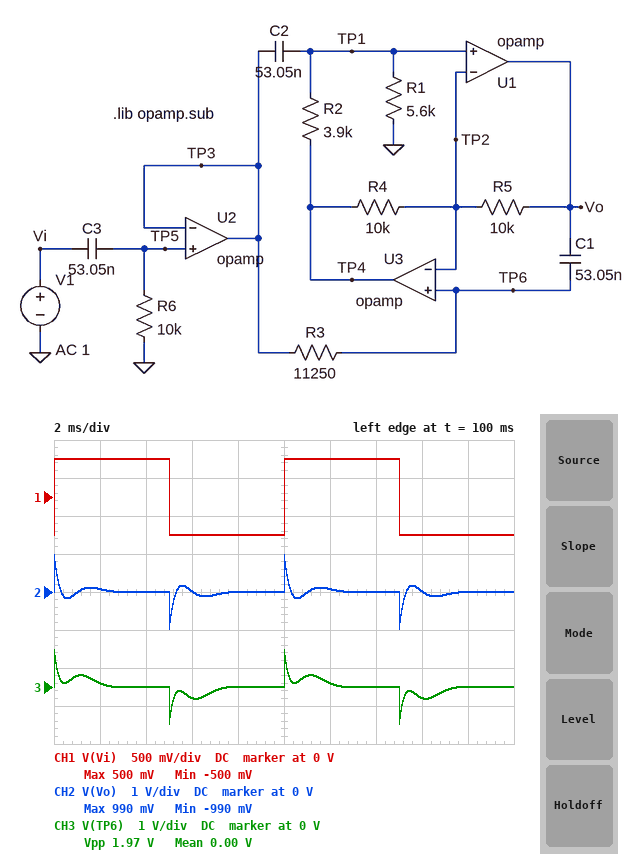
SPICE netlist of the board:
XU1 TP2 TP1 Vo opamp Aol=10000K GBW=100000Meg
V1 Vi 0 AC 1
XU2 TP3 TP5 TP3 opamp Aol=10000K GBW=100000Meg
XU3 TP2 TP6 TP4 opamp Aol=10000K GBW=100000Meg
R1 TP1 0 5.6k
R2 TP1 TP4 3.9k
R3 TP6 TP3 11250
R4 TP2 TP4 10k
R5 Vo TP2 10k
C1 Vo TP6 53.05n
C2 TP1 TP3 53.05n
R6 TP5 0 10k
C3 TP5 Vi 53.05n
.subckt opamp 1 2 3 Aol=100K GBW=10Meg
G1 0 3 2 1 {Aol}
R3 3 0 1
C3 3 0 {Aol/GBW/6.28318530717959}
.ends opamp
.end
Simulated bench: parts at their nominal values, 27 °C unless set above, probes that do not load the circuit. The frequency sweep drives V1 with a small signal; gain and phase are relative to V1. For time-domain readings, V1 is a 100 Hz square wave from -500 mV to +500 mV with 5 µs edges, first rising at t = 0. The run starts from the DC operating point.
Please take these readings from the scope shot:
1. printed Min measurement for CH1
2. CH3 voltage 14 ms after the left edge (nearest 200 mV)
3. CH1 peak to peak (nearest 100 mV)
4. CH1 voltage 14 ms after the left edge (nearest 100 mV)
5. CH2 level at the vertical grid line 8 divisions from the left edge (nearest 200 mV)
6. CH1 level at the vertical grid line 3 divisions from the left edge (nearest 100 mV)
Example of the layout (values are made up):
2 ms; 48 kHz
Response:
-500 mV; 0 V; 1.0 V; 500 mV; 0 V; -500 mV
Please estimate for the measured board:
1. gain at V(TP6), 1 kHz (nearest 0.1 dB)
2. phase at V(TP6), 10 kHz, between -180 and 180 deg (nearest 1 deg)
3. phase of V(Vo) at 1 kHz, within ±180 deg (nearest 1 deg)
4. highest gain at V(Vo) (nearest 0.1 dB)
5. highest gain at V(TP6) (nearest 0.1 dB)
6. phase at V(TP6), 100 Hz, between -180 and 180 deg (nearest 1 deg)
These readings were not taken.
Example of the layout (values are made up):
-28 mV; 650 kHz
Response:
-2.0 dB; 5 deg; 51 deg; 0 dB; 0 dB; 56 deg
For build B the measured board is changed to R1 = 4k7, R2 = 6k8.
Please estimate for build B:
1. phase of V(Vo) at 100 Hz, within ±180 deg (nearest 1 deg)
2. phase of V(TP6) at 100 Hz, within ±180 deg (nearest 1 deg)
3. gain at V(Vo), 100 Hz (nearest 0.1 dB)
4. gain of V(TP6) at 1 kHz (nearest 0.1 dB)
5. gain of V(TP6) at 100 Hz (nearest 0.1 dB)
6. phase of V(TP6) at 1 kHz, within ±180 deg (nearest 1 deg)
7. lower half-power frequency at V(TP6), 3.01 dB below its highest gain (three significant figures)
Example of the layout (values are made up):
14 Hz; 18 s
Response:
-139 deg; 41 deg; -16.0 dB; -2.2 dB; -11.3 dB; 53 deg; 859 Hz
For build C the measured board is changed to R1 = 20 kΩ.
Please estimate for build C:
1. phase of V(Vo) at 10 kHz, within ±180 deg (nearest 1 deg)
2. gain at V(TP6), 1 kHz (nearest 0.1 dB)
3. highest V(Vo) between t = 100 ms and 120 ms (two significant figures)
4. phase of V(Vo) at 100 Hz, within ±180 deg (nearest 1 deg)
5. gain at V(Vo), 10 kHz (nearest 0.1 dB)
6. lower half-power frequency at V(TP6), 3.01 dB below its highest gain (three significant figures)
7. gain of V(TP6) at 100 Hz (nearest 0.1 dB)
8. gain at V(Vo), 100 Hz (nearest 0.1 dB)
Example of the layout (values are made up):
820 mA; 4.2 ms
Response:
3 deg; -0.5 dB; 1.0 V; 67 deg; 0 dB; 564 Hz; -10.0 dB; -12.0 dB
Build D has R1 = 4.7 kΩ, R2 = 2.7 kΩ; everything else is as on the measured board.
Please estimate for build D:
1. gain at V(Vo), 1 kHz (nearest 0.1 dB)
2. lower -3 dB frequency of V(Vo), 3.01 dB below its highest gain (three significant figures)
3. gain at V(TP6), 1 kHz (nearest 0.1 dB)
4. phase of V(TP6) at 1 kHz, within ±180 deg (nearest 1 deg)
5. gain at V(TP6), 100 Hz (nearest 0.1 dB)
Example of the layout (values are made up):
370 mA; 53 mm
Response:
-1.1 dB; 718 Hz; -3.0 dB; 59 deg; -10.2 dB
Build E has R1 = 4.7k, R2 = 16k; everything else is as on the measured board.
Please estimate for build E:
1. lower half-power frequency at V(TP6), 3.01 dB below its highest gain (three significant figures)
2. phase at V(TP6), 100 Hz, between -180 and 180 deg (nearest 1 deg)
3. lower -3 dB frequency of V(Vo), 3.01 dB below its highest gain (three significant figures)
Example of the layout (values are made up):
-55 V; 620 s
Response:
798 Hz; 14 deg; 216 Hz
